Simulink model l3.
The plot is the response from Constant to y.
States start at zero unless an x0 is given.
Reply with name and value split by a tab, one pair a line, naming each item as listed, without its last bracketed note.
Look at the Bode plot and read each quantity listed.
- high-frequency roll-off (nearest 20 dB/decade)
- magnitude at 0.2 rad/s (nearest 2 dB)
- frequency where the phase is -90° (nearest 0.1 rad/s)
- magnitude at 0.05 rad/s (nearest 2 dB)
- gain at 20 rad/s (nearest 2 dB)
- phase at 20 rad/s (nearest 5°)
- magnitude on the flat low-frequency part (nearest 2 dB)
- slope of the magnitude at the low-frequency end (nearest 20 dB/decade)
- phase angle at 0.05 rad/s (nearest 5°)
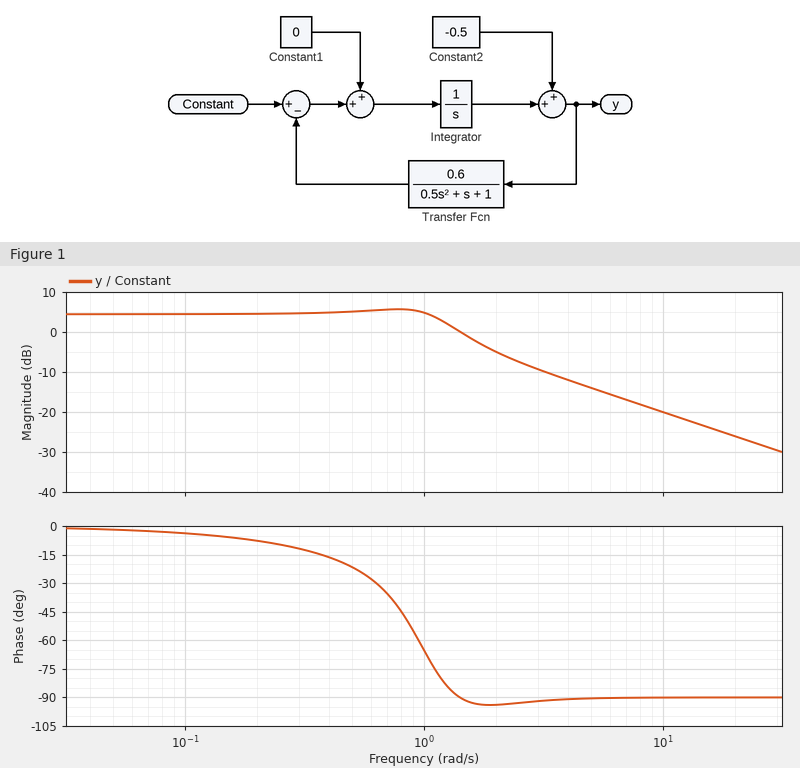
high-frequency roll-off	-20 dB/decade
magnitude at 0.2 rad/s	4 dB
frequency where the phase is -90°	1.4 rad/s
magnitude at 0.05 rad/s	4 dB
gain at 20 rad/s	-26 dB
phase at 20 rad/s	-90°
magnitude on the flat low-frequency part	4 dB
slope of the magnitude at the low-frequency end	0 dB/decade
phase angle at 0.05 rad/s	0°
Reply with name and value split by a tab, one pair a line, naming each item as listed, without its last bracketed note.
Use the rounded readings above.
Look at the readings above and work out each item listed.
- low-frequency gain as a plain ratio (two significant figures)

low-frequency gain as a plain ratio	1.6
